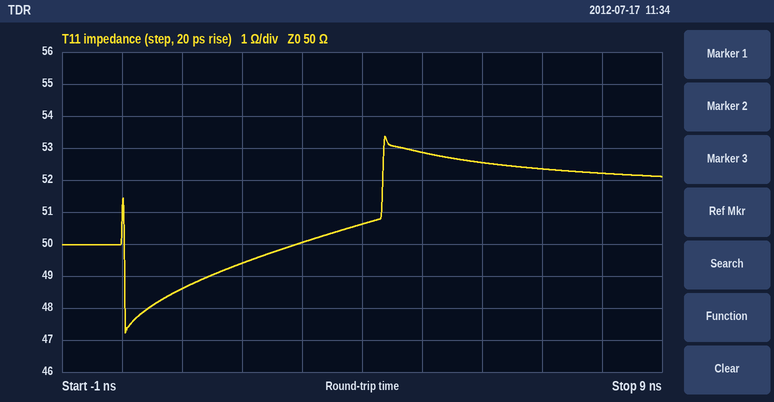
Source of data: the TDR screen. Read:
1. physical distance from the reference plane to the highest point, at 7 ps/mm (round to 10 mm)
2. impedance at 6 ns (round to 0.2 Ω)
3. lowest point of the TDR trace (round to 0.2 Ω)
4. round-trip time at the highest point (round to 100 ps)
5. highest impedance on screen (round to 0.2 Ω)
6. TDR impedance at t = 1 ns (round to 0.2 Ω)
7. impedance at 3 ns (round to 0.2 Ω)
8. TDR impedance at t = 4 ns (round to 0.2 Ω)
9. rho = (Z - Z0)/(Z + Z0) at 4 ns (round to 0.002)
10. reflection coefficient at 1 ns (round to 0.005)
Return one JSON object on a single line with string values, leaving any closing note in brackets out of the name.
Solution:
{"physical distance from the reference plane to the highest point, at 7 ps/mm": "310 mm", "impedance at 6 ns": "52.6 Ω", "lowest point of the TDR trace": "47.2 Ω", "round-trip time at the highest point": "4.4 ns", "highest impedance on screen": "53.4 Ω", "TDR impedance at t = 1 ns": "48.6 Ω", "impedance at 3 ns": "50.0 Ω", "TDR impedance at t = 4 ns": "50.6 Ω", "rho = (Z - Z0)/(Z + Z0) at 4 ns": "+0.006", "reflection coefficient at 1 ns": "-0.015"}
